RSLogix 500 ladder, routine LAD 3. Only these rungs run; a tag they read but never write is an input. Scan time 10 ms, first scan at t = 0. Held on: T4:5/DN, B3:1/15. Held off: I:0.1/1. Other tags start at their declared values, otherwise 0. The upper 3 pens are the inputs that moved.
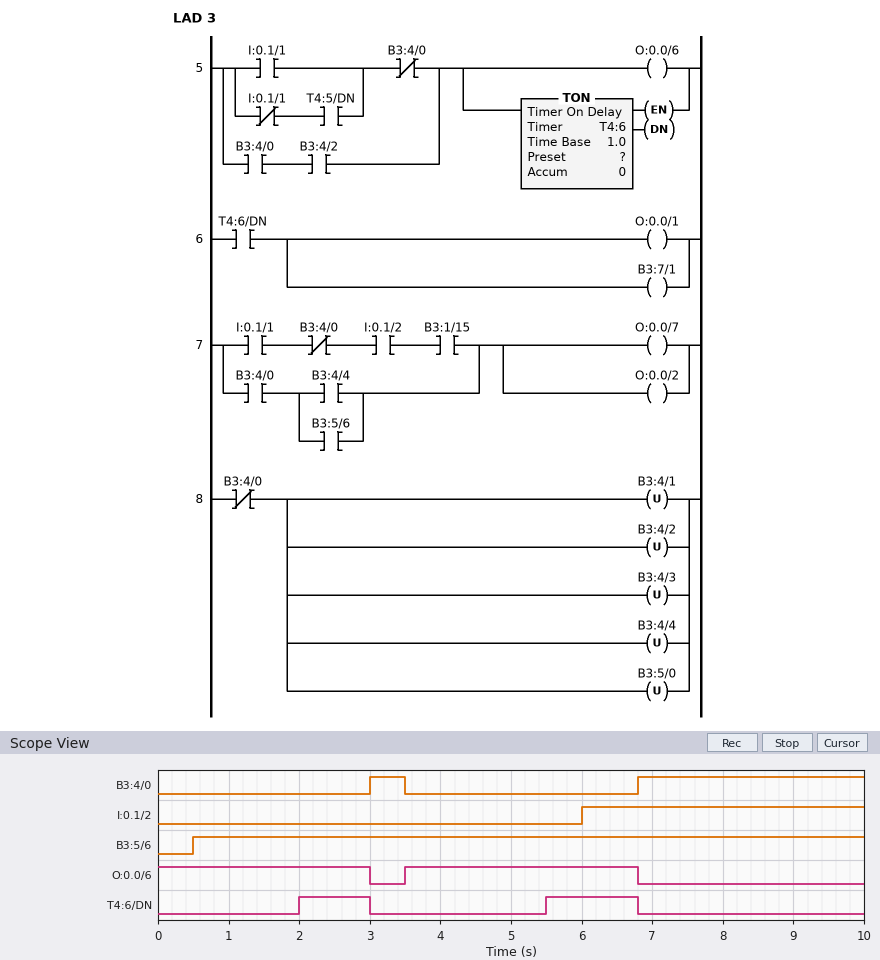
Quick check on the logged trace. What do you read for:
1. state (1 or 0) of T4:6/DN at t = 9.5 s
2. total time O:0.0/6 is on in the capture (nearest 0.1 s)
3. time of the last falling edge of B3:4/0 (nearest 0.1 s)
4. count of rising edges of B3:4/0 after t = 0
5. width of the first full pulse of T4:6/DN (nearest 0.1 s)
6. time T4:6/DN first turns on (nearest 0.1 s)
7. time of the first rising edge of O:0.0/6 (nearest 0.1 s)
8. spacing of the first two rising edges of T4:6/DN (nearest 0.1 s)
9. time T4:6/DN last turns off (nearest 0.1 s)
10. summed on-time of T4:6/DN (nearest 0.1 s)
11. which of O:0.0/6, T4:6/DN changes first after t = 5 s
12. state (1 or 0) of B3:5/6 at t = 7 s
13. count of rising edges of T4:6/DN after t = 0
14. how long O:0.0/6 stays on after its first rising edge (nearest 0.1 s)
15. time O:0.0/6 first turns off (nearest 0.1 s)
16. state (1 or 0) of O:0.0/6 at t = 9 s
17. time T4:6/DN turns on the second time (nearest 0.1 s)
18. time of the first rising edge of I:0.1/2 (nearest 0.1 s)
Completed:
0
6.3 s
3.5 s
2
1.0 s
2.0 s
3.5 s
3.5 s
6.8 s
2.3 s
T4:6/DN
1
2
3.3 s
3.0 s
0
5.5 s
6.0 s
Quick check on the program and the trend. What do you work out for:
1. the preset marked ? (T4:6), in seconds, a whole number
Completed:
2 s
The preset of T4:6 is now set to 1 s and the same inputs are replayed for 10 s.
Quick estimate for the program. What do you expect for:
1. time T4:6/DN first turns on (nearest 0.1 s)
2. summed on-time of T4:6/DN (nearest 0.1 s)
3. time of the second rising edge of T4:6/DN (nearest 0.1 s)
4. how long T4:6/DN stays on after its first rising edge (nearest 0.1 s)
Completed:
1.0 s
4.3 s
4.5 s
2.0 s
